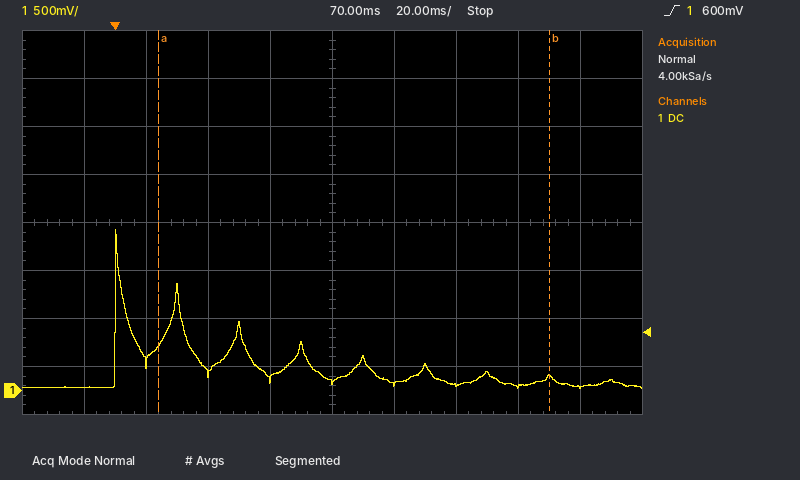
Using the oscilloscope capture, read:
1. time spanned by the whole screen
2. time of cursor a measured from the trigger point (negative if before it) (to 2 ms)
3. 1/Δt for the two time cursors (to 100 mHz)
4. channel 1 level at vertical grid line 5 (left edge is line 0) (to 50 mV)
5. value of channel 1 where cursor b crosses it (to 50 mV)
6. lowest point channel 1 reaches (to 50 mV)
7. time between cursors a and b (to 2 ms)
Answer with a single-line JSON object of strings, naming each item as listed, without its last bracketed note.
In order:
{"time spanned by the whole screen": "200 ms", "time of cursor a measured from the trigger point (negative if before it)": "+14 ms", "1/Δt for the two time cursors": "7.9 Hz", "channel 1 level at vertical grid line 5 (left edge is line 0)": "100 mV", "value of channel 1 where cursor b crosses it": "150 mV", "lowest point channel 1 reaches": "0 mV", "time between cursors a and b": "126 ms"}
